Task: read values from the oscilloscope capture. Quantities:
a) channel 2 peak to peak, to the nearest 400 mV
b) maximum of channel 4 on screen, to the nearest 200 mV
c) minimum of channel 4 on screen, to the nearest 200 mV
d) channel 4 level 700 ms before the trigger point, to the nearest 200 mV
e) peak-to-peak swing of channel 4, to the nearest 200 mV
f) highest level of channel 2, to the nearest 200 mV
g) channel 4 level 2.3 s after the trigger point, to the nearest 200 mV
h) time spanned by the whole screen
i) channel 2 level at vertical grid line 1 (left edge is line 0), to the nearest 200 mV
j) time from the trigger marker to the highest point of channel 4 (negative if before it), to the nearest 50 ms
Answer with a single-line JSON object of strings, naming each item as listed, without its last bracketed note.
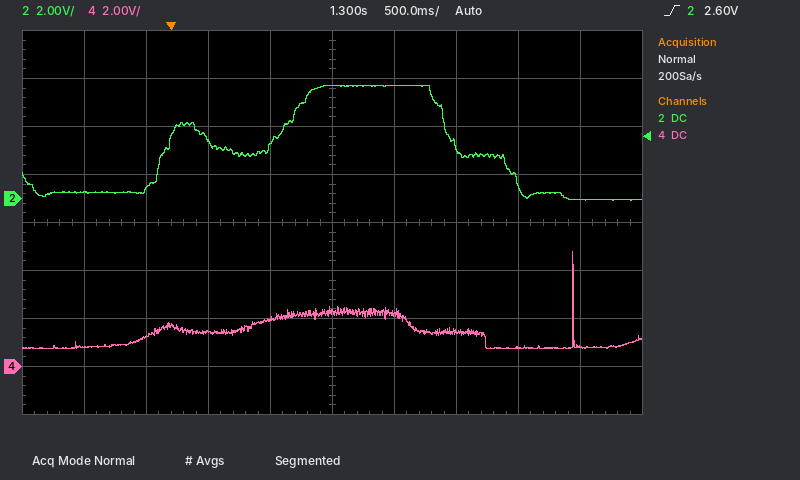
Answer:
{"channel 2 peak to peak, to the nearest 400 mV": "4.8 V", "maximum of channel 4 on screen, to the nearest 200 mV": "4.8 V", "minimum of channel 4 on screen, to the nearest 200 mV": "800 mV", "channel 4 level 700 ms before the trigger point, to the nearest 200 mV": "800 mV", "peak-to-peak swing of channel 4, to the nearest 200 mV": "4.0 V", "highest level of channel 2, to the nearest 200 mV": "4.8 V", "channel 4 level 2.3 s after the trigger point, to the nearest 200 mV": "1.4 V", "time spanned by the whole screen": "5 s", "channel 2 level at vertical grid line 1 (left edge is line 0), to the nearest 200 mV": "200 mV", "time from the trigger marker to the highest point of channel 4 (negative if before it), to the nearest 50 ms": "+3.25 s"}
